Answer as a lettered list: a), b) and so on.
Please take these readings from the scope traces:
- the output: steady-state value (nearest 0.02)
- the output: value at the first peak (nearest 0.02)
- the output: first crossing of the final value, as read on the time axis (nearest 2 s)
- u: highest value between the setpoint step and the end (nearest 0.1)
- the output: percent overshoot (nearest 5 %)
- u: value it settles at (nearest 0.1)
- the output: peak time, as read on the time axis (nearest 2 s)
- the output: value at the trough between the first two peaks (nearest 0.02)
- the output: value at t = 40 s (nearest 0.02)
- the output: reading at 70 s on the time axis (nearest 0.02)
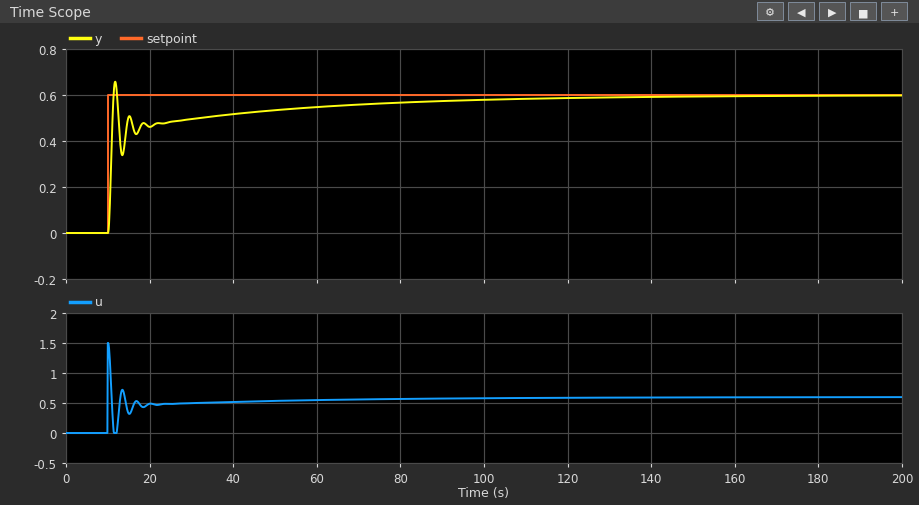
a) 0.60
b) 0.66
c) 12 s
d) 1.5
e) 10 %
f) 0.6
g) 12 s
h) 0.34
i) 0.52
j) 0.56
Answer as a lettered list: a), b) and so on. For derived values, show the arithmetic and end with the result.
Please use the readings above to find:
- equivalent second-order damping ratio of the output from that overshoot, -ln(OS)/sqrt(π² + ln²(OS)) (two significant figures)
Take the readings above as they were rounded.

a) ln(0.1) = -2.303; 2.303 / sqrt(9.870 + 5.302) = 0.59
